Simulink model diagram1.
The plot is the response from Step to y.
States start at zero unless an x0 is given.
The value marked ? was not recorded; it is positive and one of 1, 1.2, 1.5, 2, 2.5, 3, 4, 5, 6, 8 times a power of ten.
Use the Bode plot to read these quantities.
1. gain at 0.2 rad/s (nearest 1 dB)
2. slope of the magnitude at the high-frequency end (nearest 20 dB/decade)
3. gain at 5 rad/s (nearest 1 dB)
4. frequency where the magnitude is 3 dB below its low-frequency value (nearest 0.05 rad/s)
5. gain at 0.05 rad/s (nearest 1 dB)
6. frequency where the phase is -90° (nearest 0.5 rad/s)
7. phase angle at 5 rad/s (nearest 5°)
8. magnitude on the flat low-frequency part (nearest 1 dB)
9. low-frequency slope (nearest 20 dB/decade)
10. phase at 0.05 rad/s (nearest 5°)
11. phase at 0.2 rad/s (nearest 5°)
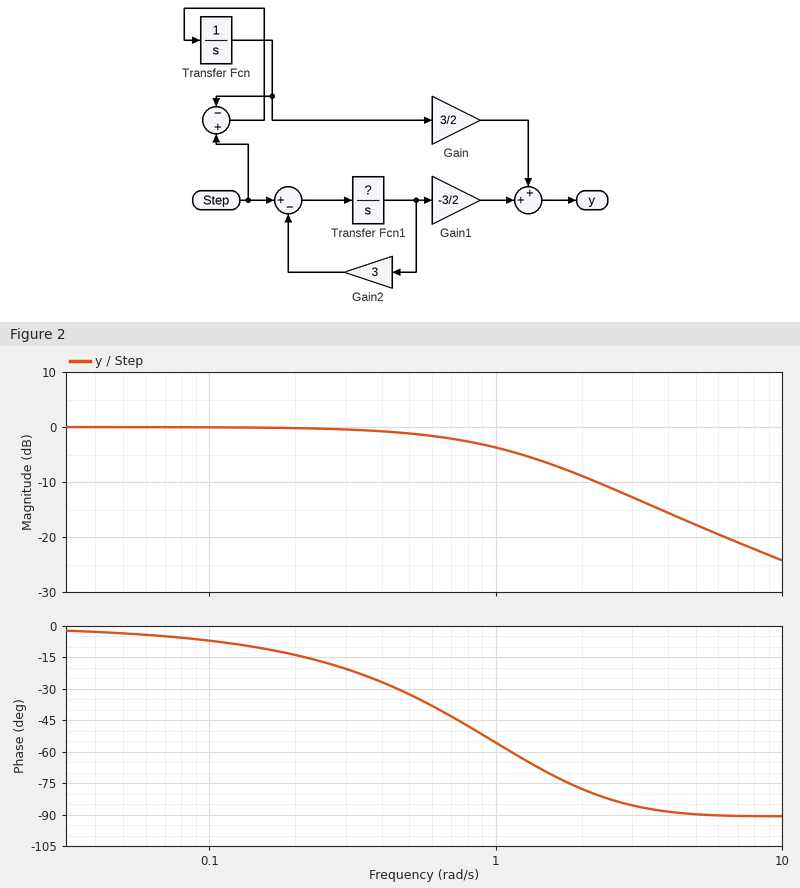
0 dB
-20 dB/decade
-18 dB
0.85 rad/s
0 dB
5.0 rad/s
-90°
0 dB
0 dB/decade
-5°
-15°
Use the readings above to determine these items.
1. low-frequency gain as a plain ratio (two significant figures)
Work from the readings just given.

1.0
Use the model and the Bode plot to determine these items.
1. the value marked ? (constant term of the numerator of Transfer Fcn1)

0.6
